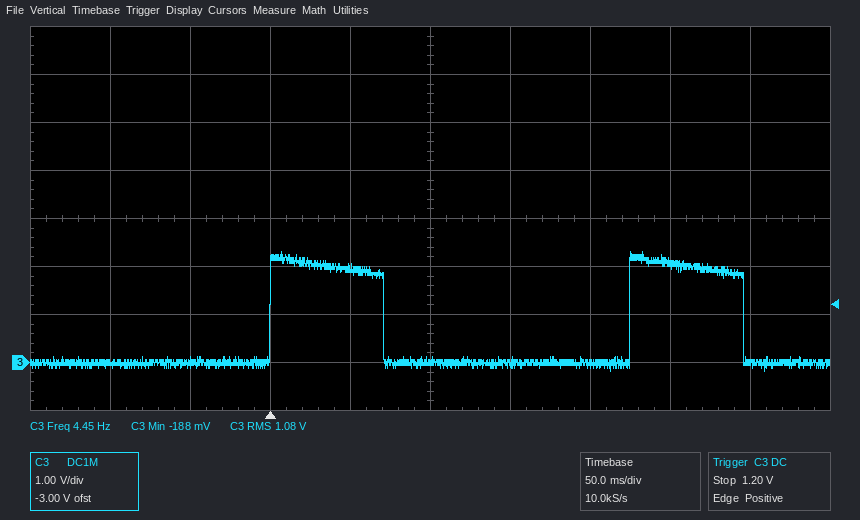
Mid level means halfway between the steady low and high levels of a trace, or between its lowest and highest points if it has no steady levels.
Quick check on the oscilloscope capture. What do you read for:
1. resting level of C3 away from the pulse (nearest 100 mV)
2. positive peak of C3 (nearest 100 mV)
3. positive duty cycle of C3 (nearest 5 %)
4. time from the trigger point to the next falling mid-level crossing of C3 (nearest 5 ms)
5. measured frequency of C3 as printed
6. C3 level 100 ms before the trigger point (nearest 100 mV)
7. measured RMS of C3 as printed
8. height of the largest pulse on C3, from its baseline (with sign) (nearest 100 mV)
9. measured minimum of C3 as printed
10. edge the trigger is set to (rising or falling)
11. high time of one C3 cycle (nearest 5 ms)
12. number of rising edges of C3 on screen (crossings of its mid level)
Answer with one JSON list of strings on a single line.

["0.0 V", "2.3 V", "30 %", "70 ms", "4.45 Hz", "0.0 V", "1.08 V", "+2.3 V", "-188 mV", "rising", "70 ms", "2"]
